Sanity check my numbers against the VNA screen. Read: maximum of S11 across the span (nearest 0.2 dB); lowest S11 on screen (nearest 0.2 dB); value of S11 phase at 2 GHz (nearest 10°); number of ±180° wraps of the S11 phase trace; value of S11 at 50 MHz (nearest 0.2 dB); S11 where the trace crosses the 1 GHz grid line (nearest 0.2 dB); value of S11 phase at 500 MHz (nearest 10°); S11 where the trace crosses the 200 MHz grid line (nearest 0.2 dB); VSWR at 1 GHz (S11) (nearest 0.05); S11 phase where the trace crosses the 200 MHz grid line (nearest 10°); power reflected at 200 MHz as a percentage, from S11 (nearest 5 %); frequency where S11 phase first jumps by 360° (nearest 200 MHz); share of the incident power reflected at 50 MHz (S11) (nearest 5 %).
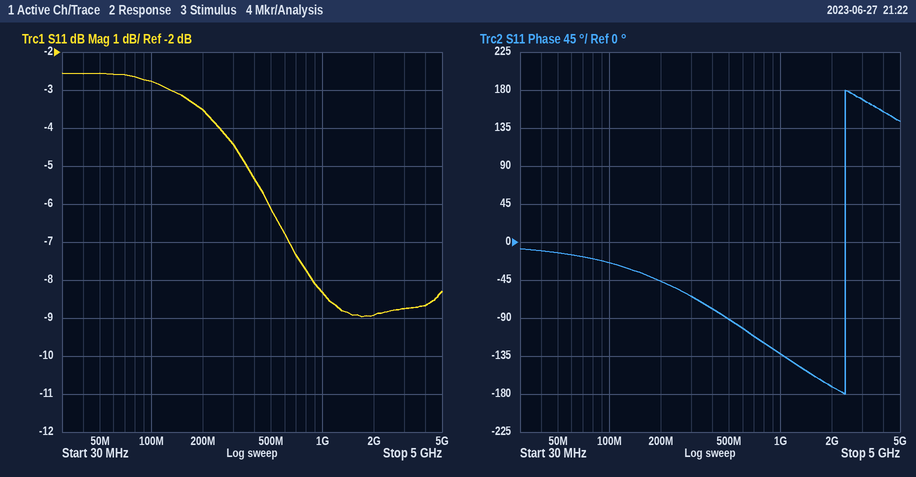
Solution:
-2.6 dB
-9.0 dB
-170°
1
-2.6 dB
-8.4 dB
-90°
-3.6 dB
2.25
-50°
45 %
2.4 GHz
55 %
